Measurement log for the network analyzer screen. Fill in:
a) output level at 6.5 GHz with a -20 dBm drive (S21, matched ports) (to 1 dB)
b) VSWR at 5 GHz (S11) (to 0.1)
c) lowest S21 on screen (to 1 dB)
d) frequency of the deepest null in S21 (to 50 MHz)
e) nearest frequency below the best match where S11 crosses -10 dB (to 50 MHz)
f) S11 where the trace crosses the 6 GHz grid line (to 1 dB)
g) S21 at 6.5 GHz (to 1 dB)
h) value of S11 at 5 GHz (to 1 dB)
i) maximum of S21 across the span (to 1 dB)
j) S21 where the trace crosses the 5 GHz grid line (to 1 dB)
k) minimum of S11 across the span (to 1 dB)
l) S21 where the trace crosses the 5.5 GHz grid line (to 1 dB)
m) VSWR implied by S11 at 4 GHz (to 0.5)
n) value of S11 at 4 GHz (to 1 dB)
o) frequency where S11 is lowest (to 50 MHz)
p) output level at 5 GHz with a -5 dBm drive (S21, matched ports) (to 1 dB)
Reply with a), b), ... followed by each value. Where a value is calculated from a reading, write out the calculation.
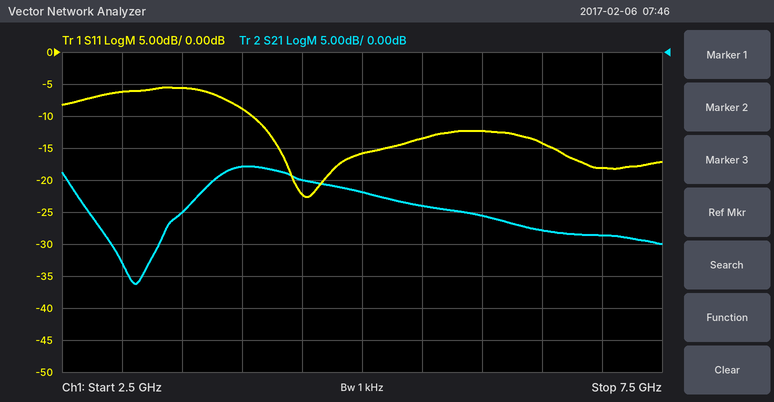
a) -20 dBm + (-28 dB) = -48 dBm
b) |Γ| = 10^(-16/20) = 0.1585; VSWR = (1 + 0.1585)/(1 − 0.1585) ≈ 1.4
c) -36 dB
d) 3.10 GHz
e) 4.10 GHz
f) -12 dB
g) -28 dB
h) -16 dB
i) -18 dB
j) -22 dB
k) -23 dB
l) -24 dB
m) |Γ| = 10^(-9/20) = 0.3548; VSWR = (1 + 0.3548)/(1 − 0.3548) ≈ 2.10, so 2.0 to the nearest 0.5
n) -9 dB
o) 4.55 GHz
p) -5 dBm + (-22 dB) = -27 dBm
